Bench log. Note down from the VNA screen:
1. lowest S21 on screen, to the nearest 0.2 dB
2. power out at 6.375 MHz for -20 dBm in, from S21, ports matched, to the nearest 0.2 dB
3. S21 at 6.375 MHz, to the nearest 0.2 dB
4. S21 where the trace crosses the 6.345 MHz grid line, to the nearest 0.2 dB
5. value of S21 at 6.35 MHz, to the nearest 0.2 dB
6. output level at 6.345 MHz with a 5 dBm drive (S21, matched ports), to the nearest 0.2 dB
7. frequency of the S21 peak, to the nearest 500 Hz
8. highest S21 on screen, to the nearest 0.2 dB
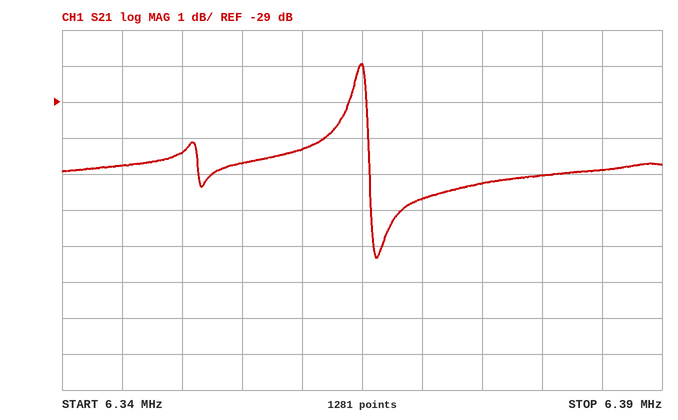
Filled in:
-33.4 dB
-51.2 dBm
-31.2 dB
-30.8 dB
-30.4 dB
-25.8 dBm
6.3650 MHz
-28.0 dB
